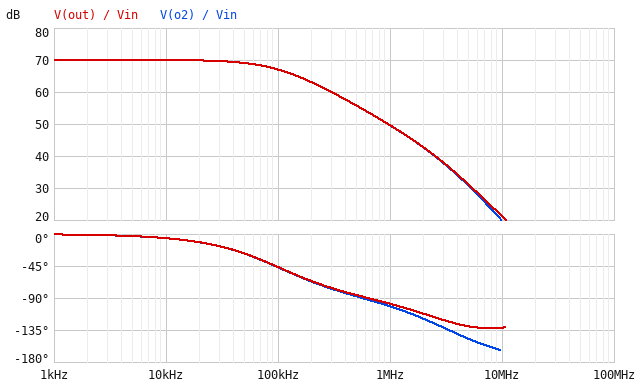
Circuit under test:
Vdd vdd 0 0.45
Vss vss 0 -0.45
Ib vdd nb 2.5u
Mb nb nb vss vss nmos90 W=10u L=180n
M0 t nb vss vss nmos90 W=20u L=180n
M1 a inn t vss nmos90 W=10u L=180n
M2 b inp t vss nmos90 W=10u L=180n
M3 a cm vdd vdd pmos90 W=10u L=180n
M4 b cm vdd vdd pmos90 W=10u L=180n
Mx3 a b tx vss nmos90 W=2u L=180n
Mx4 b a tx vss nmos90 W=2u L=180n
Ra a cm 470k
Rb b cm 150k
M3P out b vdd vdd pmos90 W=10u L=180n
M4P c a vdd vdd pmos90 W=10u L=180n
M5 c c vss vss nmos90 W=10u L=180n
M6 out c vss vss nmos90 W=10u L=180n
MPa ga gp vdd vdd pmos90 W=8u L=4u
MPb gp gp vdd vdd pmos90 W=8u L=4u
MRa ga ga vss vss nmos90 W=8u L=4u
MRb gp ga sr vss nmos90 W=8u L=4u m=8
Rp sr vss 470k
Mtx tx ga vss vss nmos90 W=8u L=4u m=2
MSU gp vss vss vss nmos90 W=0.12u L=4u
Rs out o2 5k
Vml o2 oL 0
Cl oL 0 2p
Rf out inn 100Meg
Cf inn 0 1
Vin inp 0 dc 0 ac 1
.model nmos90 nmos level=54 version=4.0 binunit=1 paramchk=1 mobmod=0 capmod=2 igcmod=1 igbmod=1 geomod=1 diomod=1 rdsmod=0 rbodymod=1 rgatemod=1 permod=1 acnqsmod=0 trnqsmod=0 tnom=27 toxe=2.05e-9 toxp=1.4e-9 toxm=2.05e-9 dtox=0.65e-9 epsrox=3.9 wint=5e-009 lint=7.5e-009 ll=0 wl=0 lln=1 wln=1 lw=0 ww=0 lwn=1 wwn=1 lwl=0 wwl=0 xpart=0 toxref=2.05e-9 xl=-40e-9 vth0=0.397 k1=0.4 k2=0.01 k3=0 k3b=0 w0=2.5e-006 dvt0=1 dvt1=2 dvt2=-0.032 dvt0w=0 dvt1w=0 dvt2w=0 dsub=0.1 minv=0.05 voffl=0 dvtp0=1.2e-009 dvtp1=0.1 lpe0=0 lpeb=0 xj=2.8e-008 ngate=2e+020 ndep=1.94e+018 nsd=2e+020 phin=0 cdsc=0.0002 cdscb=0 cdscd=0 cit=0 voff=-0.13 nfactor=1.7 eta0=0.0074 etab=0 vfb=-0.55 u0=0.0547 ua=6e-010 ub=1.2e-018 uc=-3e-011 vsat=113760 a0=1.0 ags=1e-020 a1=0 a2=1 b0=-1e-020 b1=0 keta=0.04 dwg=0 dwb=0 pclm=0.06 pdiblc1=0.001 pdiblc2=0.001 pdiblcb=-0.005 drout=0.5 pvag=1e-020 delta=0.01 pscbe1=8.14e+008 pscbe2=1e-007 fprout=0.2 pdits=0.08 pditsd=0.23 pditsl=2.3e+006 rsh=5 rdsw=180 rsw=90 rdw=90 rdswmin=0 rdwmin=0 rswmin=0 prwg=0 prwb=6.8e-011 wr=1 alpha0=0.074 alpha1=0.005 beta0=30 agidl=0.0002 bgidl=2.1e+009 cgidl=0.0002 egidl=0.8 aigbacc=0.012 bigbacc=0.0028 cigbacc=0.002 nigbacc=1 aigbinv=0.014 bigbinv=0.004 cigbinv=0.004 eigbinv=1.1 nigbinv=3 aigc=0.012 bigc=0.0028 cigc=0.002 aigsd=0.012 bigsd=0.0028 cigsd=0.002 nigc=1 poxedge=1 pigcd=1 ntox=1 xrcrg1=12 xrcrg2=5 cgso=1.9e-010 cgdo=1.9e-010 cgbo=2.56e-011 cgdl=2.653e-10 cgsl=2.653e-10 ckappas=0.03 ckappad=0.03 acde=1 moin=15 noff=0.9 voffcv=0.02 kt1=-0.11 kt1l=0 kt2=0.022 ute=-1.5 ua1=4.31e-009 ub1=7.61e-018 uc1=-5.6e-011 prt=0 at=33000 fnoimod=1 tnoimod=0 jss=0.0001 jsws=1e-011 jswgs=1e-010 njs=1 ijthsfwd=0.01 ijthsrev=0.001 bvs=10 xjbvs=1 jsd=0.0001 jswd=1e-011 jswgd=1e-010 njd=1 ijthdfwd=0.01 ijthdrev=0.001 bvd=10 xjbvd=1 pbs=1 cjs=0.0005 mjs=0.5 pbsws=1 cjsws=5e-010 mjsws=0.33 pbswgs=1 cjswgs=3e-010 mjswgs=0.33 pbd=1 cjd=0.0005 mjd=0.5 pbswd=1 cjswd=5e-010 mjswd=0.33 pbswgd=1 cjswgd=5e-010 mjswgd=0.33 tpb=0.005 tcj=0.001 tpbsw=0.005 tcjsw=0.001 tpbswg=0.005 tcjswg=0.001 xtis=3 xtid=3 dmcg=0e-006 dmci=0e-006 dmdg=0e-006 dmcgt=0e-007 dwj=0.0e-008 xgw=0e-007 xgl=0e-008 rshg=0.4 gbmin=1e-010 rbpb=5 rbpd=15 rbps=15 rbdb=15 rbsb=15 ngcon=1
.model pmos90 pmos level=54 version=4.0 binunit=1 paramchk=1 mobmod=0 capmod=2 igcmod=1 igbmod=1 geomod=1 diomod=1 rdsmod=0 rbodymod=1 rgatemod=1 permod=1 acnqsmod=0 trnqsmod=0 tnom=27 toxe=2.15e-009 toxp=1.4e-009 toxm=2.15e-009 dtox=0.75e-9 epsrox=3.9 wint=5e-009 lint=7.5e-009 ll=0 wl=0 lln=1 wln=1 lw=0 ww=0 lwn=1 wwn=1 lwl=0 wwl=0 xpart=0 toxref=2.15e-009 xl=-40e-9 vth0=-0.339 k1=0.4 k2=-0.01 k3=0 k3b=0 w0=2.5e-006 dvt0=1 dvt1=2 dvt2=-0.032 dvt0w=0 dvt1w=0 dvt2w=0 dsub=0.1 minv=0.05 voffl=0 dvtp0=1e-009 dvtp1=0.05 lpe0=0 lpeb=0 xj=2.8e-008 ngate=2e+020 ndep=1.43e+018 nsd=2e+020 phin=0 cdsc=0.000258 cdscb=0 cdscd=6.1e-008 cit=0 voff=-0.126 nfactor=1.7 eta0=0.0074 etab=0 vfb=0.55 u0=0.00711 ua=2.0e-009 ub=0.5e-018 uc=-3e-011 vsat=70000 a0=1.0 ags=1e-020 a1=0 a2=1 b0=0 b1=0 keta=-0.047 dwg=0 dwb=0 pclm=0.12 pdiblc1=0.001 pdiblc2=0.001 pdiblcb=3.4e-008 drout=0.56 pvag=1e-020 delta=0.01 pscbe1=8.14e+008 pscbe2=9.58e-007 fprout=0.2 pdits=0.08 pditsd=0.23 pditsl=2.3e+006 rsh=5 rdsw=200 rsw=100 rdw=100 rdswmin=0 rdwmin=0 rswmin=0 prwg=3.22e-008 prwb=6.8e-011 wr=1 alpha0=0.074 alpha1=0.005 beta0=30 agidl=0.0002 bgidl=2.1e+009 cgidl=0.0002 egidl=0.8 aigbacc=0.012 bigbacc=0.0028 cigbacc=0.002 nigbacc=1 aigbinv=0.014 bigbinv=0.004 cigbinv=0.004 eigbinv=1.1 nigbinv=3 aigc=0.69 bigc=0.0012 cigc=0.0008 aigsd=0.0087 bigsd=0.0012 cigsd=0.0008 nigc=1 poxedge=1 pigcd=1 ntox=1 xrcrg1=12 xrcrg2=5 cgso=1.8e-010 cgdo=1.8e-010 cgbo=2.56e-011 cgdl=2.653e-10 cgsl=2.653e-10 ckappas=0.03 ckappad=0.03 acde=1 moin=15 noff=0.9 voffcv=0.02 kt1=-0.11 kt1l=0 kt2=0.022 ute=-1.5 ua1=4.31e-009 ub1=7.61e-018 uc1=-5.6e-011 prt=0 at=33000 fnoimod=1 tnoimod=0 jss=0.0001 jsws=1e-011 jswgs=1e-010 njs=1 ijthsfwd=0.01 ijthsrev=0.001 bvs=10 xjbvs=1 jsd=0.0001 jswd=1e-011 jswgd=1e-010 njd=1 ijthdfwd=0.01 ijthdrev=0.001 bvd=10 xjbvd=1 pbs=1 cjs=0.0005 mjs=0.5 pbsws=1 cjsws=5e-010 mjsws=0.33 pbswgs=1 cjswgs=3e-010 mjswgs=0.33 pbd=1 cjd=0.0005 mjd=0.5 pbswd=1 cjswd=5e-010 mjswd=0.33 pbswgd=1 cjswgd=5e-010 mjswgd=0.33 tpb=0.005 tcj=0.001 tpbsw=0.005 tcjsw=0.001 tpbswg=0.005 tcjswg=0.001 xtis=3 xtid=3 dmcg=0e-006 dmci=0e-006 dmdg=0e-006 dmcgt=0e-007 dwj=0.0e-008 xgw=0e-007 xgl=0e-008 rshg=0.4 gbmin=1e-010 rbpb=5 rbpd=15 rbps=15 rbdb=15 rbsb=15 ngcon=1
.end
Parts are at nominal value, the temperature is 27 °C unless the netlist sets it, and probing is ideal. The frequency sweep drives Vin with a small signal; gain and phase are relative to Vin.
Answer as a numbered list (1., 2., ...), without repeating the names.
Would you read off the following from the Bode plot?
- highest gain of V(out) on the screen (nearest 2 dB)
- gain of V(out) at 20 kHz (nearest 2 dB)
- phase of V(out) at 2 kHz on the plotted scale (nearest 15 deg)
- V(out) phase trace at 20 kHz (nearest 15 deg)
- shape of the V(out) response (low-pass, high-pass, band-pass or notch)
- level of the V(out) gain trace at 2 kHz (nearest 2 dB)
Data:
1. 70 dB
2. 70 dB
3. 0 deg
4. -15 deg
5. low-pass
6. 70 dB
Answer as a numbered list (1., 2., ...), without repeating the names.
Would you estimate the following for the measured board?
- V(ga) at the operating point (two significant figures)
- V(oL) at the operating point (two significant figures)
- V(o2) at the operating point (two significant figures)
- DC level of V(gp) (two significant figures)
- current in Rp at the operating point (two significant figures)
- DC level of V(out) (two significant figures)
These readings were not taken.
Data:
1. -180 mV
2. 1.6 mV
3. 1.6 mV
4. 120 mV
5. 150 nA
6. 1.6 mV
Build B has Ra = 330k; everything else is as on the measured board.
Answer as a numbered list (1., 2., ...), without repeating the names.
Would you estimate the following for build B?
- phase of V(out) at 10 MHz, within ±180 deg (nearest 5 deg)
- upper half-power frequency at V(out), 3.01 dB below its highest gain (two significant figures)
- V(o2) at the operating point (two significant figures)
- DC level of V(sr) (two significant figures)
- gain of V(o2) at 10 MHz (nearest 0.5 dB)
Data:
1. -115 deg
2. 110 kHz
3. 1.5 mV
4. -380 mV
5. 19.0 dB
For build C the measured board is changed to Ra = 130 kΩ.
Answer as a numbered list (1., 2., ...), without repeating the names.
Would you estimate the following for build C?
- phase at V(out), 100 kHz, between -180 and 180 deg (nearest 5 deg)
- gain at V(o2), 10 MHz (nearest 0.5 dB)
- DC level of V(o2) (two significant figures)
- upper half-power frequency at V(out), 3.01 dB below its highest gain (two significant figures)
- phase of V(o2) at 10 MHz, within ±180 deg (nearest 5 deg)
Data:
1. -40 deg
2. 14.5 dB
3. 1.2 mV
4. 120 kHz
5. -120 deg
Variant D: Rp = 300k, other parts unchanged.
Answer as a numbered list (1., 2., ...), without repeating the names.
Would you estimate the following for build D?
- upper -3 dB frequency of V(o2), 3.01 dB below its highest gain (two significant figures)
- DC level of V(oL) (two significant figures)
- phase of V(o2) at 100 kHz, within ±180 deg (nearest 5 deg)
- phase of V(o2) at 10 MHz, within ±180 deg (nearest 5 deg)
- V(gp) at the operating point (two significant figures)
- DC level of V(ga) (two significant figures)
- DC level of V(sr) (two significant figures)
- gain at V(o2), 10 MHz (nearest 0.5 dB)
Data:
1. 130 kHz
2. 1.8 mV
3. 145 deg
4. 155 deg
5. 100 mV
6. -160 mV
7. -380 mV
8. 19.5 dB
